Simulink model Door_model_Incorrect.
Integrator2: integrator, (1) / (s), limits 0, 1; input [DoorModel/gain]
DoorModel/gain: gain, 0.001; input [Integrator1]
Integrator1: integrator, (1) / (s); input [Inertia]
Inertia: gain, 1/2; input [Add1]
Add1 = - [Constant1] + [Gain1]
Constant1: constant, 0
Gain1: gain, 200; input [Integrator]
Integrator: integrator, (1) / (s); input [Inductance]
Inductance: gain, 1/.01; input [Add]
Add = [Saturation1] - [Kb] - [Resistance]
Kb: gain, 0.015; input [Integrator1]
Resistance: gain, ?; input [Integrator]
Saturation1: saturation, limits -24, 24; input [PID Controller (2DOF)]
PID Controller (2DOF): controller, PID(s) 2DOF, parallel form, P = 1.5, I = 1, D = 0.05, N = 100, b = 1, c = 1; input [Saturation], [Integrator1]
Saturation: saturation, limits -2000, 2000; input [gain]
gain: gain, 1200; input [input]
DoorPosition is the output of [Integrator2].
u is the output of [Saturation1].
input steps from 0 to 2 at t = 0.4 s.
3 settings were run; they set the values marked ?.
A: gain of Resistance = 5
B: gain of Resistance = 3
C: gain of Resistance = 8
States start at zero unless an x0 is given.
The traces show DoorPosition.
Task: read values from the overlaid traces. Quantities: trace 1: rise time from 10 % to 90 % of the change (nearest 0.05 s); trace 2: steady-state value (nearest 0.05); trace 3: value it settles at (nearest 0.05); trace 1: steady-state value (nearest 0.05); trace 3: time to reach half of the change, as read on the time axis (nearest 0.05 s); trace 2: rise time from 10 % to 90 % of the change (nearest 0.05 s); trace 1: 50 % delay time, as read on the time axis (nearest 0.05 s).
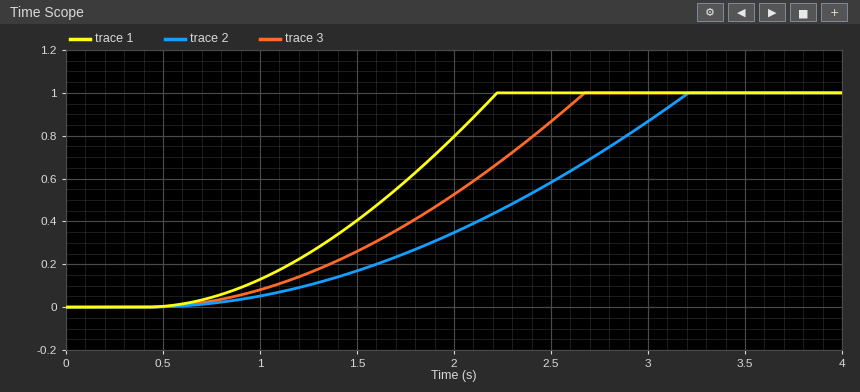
1.20 s
1.00
1.00
1.00
1.95 s
1.80 s
1.65 s
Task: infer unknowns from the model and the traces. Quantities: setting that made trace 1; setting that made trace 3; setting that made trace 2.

B
A
C
